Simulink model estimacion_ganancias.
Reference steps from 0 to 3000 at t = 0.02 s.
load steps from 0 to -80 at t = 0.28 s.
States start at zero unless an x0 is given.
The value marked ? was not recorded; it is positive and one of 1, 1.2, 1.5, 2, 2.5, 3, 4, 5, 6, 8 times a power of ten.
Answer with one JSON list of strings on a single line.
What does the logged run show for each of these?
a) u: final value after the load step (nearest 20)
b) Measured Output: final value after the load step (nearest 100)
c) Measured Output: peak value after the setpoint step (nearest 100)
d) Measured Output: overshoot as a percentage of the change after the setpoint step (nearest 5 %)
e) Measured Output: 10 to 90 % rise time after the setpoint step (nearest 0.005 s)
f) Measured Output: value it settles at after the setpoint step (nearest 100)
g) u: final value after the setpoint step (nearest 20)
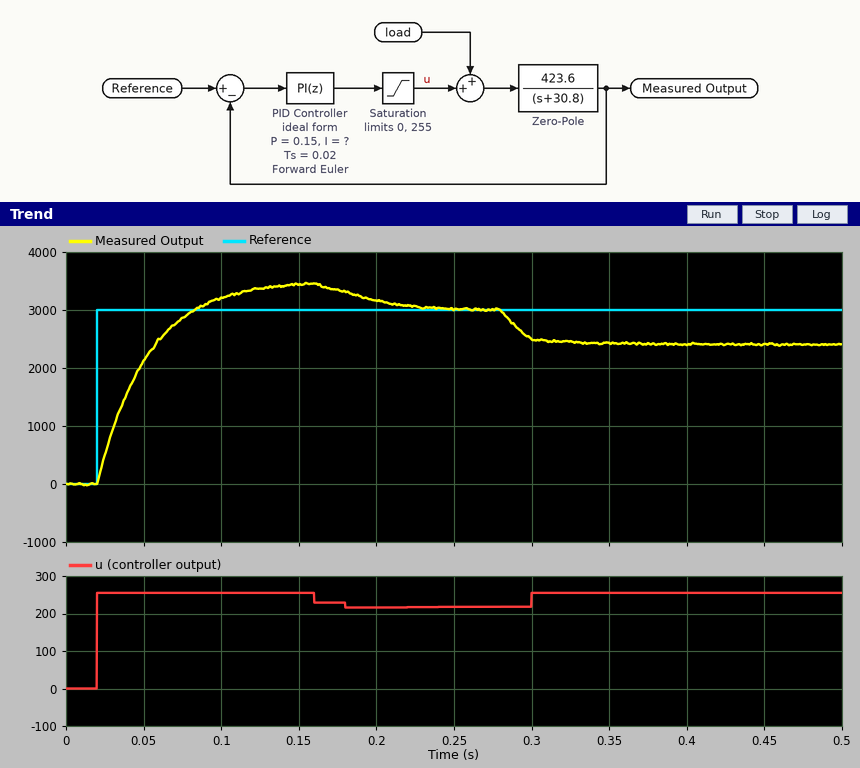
["260", "2400", "3500", "15 %", "0.045 s", "3000", "220"]
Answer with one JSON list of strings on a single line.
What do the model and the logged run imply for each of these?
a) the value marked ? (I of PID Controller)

["25"]
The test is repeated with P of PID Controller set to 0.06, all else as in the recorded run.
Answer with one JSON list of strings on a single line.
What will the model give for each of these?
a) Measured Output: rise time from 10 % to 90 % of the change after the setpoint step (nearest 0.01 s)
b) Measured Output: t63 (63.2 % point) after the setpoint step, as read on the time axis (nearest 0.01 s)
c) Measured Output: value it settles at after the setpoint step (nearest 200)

["0.08 s", "0.06 s", "3000"]
